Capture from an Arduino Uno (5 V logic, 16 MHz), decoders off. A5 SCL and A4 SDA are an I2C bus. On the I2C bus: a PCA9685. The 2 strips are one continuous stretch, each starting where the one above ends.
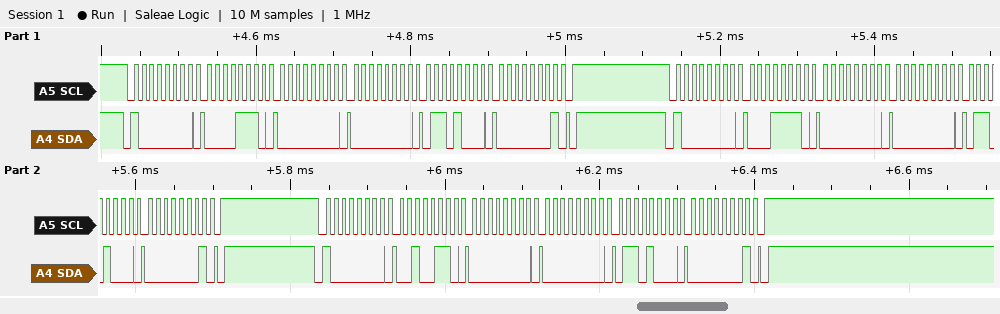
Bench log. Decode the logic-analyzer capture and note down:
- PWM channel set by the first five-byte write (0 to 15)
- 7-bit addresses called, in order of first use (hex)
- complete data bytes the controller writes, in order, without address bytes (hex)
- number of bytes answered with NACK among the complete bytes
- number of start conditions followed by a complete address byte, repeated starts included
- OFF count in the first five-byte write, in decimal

2
0x40
0E 00 00 68 01 1E 00 00 68 01 26 00 00 68 01
0
3
360
